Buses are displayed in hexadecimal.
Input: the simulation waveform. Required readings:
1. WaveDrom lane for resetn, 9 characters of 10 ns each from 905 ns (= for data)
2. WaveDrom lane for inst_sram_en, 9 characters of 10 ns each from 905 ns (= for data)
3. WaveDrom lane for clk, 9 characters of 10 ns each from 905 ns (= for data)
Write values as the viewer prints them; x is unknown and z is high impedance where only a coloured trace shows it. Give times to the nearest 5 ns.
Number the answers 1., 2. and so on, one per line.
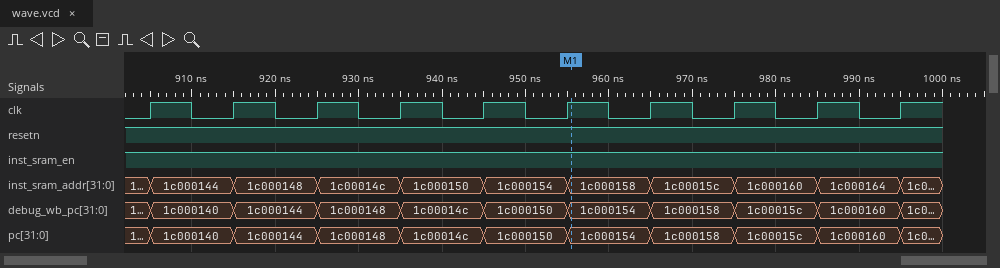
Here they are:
1. {name: 'resetn', wave: '1........'}
2. {name: 'inst_sram_en', wave: '1........'}
3. {name: 'clk', wave: 'p........'}
